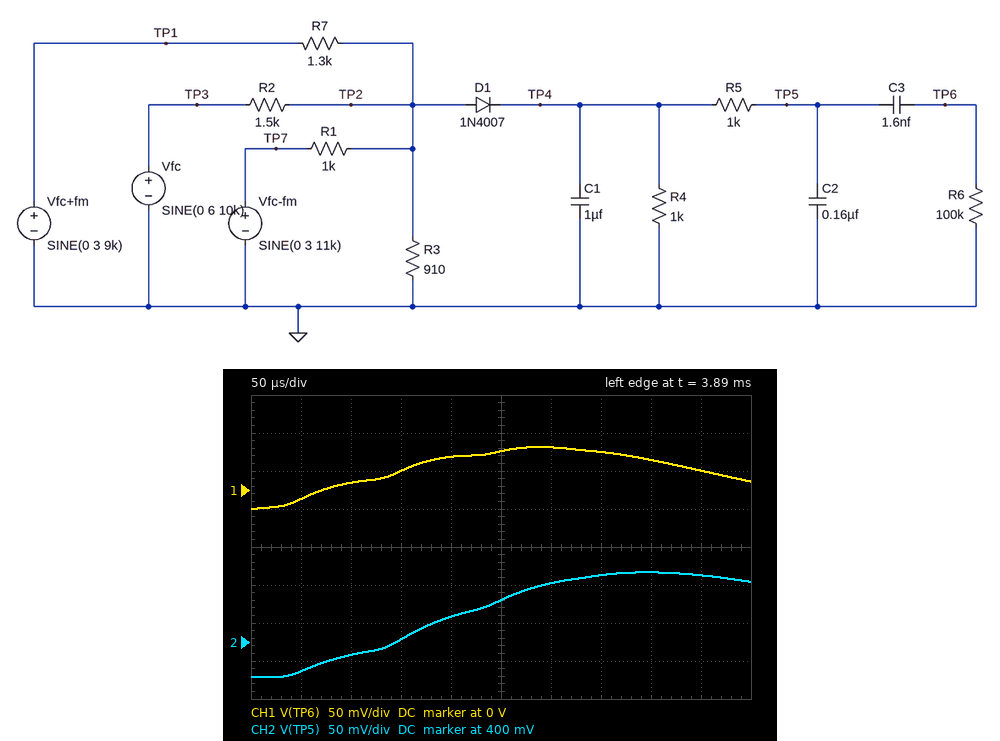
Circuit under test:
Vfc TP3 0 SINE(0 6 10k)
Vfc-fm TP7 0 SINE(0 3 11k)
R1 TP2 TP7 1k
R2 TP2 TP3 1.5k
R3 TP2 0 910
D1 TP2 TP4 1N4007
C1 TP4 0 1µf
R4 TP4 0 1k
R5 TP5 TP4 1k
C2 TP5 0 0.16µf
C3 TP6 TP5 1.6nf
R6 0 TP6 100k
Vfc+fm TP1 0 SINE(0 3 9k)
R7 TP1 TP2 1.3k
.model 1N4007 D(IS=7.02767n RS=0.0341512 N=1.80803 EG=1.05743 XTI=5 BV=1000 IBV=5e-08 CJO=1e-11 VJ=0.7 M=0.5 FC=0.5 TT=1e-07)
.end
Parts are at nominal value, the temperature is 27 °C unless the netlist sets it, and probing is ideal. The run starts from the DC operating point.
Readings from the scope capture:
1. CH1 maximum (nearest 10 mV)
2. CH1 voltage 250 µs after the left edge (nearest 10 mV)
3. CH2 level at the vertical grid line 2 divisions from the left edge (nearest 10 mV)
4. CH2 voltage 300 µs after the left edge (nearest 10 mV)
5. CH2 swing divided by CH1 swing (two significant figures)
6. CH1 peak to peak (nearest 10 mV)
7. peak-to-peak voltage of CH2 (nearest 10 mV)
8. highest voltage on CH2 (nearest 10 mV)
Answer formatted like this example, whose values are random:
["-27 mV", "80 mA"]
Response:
["60 mV", "50 mV", "380 mV", "480 mV", "1.7", "80 mV", "140 mV", "490 mV"]
